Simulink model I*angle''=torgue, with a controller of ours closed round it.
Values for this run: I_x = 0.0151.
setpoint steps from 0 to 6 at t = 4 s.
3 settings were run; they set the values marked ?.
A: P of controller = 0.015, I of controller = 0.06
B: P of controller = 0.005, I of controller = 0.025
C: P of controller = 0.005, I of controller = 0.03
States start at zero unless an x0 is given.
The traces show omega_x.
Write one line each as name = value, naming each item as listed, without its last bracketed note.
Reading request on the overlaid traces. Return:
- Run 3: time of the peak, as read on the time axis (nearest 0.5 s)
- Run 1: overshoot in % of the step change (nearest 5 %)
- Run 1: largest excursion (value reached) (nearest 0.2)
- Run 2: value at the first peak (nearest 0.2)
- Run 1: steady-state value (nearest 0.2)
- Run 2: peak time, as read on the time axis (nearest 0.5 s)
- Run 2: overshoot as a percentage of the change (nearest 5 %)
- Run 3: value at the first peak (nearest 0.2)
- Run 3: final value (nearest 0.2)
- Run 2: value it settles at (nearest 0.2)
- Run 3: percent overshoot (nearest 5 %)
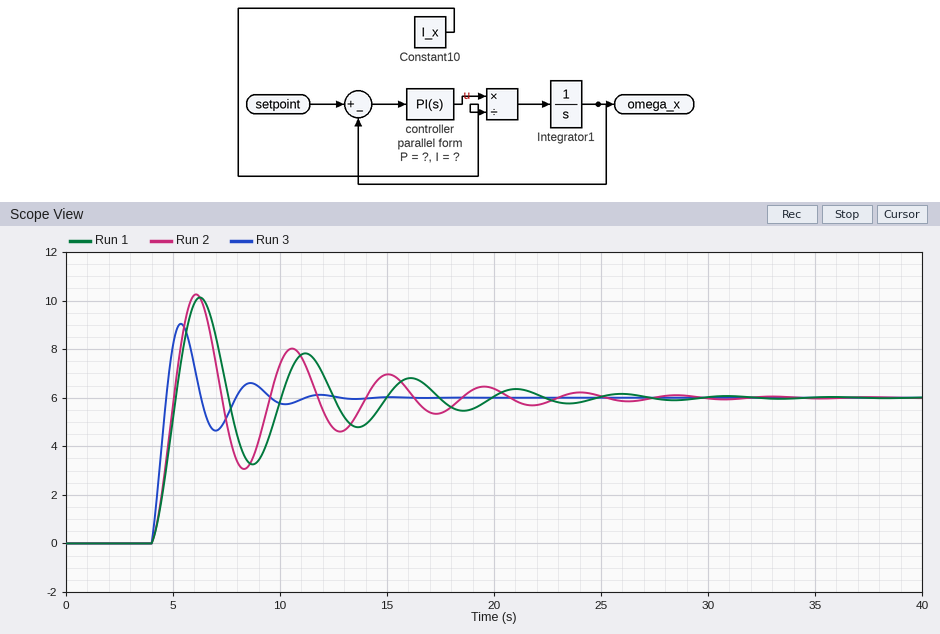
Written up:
Run 3: time of the peak, as read on the time axis = 5.5 s
Run 1: overshoot in % of the step change = 70 %
Run 1: largest excursion (value reached) = 10.2
Run 2: value at the first peak = 10.2
Run 1: steady-state value = 6.0
Run 2: peak time, as read on the time axis = 6.0 s
Run 2: overshoot as a percentage of the change = 70 %
Run 3: value at the first peak = 9.0
Run 3: final value = 6.0
Run 2: value it settles at = 6.0
Run 3: percent overshoot = 50 %
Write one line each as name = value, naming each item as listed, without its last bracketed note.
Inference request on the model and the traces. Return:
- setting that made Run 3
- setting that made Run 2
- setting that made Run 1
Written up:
setting that made Run 3 = A
setting that made Run 2 = C
setting that made Run 1 = B
